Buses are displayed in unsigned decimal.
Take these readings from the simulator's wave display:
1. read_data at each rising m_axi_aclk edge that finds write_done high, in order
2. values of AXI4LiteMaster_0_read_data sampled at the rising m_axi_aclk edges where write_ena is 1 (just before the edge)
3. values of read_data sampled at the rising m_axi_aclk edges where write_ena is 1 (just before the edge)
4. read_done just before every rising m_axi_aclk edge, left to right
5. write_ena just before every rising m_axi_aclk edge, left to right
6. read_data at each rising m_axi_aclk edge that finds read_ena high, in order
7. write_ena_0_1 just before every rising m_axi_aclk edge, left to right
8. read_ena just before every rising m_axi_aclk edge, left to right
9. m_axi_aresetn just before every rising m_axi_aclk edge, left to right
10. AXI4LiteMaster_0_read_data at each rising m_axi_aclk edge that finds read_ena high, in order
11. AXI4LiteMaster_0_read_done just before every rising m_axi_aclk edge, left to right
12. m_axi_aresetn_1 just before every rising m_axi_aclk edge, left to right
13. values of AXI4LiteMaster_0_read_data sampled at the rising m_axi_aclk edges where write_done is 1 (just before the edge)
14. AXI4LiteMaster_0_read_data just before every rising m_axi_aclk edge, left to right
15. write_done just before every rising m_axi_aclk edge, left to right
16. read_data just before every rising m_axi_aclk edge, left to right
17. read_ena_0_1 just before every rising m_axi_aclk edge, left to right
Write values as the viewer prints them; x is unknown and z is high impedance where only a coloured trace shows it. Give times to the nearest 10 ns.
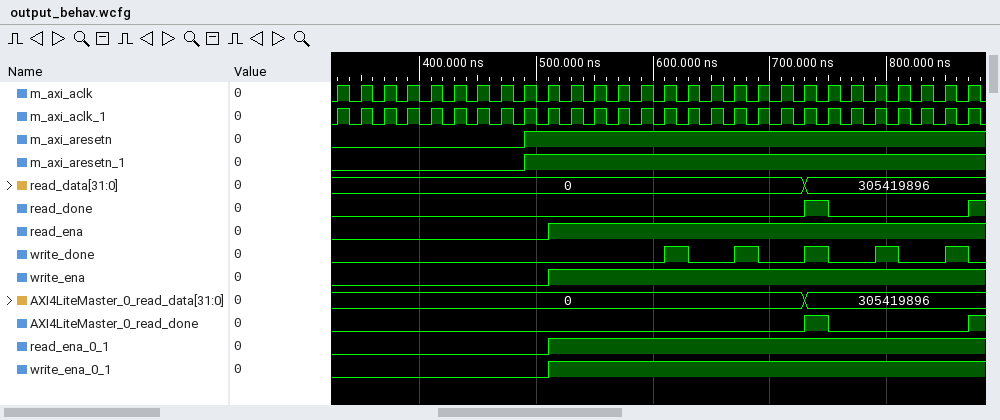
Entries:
0, 0, 305419896, 305419896, 305419896
0, 0, 0, 0, 0, 0, 0, 0, 0, 0, 0, 305419896, 305419896, 305419896, 305419896, 305419896, 305419896, 305419896
0, 0, 0, 0, 0, 0, 0, 0, 0, 0, 0, 305419896, 305419896, 305419896, 305419896, 305419896, 305419896, 305419896
0 0 0 0 0 0 0 0 0 0 0 0 0 0 0 0 0 0 0 0 0 1 0 0 0 0 0 0
0 0 0 0 0 0 0 0 0 0 1 1 1 1 1 1 1 1 1 1 1 1 1 1 1 1 1 1
0, 0, 0, 0, 0, 0, 0, 0, 0, 0, 0, 305419896, 305419896, 305419896, 305419896, 305419896, 305419896, 305419896
0 0 0 0 0 0 0 0 0 0 1 1 1 1 1 1 1 1 1 1 1 1 1 1 1 1 1 1
0 0 0 0 0 0 0 0 0 0 1 1 1 1 1 1 1 1 1 1 1 1 1 1 1 1 1 1
0 0 0 0 0 0 0 0 0 1 1 1 1 1 1 1 1 1 1 1 1 1 1 1 1 1 1 1
0, 0, 0, 0, 0, 0, 0, 0, 0, 0, 0, 305419896, 305419896, 305419896, 305419896, 305419896, 305419896, 305419896
0 0 0 0 0 0 0 0 0 0 0 0 0 0 0 0 0 0 0 0 0 1 0 0 0 0 0 0
0 0 0 0 0 0 0 0 0 1 1 1 1 1 1 1 1 1 1 1 1 1 1 1 1 1 1 1
0, 0, 305419896, 305419896, 305419896
0, 0, 0, 0, 0, 0, 0, 0, 0, 0, 0, 0, 0, 0, 0, 0, 0, 0, 0, 0, 0, 305419896, 305419896, 305419896, 305419896, 305419896, 305419896, 305419896
0 0 0 0 0 0 0 0 0 0 0 0 0 0 0 1 0 0 1 0 0 1 0 0 1 0 0 1
0, 0, 0, 0, 0, 0, 0, 0, 0, 0, 0, 0, 0, 0, 0, 0, 0, 0, 0, 0, 0, 305419896, 305419896, 305419896, 305419896, 305419896, 305419896, 305419896
0 0 0 0 0 0 0 0 0 0 1 1 1 1 1 1 1 1 1 1 1 1 1 1 1 1 1 1
